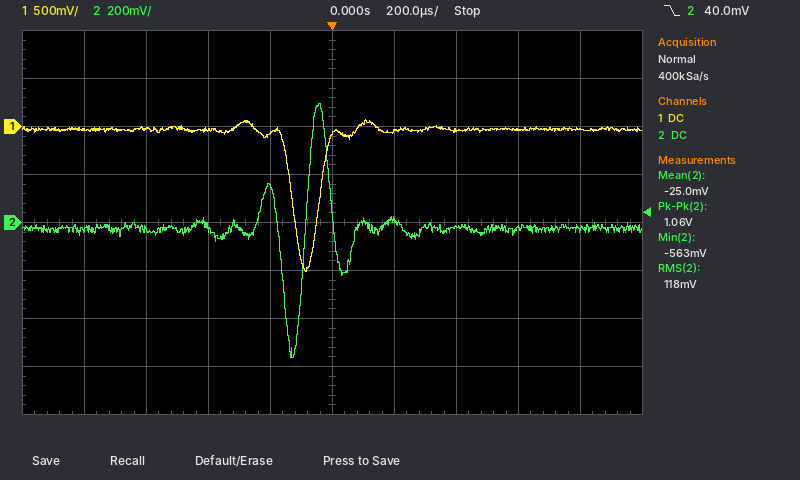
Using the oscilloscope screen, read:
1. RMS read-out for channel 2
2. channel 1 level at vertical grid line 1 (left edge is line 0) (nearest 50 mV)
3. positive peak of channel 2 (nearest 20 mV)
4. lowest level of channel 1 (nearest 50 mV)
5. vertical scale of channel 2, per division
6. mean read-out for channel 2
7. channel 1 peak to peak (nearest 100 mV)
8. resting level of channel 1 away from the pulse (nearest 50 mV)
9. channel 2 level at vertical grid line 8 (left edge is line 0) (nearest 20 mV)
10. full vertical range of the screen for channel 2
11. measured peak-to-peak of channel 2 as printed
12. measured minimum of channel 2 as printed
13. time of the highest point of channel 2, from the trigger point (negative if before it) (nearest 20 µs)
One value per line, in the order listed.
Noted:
118 mV
-50 mV
500 mV
-1.50 V
200 mV
-25.0 mV
1.60 V
-50 mV
-20 mV
1.6 V
1.06 V
-563 mV
-40 µs
